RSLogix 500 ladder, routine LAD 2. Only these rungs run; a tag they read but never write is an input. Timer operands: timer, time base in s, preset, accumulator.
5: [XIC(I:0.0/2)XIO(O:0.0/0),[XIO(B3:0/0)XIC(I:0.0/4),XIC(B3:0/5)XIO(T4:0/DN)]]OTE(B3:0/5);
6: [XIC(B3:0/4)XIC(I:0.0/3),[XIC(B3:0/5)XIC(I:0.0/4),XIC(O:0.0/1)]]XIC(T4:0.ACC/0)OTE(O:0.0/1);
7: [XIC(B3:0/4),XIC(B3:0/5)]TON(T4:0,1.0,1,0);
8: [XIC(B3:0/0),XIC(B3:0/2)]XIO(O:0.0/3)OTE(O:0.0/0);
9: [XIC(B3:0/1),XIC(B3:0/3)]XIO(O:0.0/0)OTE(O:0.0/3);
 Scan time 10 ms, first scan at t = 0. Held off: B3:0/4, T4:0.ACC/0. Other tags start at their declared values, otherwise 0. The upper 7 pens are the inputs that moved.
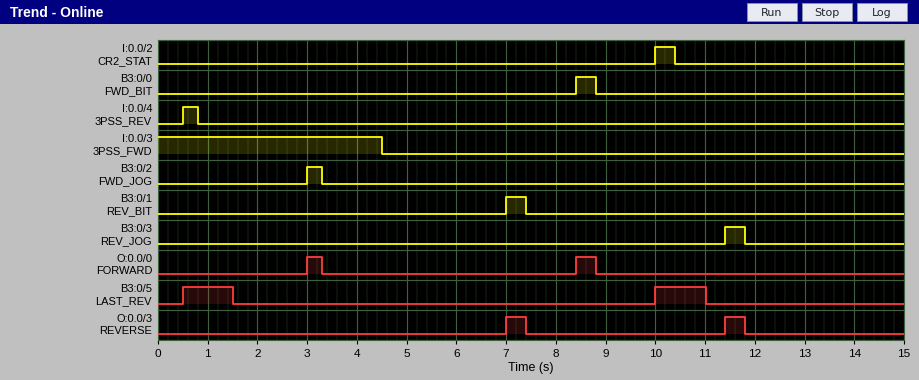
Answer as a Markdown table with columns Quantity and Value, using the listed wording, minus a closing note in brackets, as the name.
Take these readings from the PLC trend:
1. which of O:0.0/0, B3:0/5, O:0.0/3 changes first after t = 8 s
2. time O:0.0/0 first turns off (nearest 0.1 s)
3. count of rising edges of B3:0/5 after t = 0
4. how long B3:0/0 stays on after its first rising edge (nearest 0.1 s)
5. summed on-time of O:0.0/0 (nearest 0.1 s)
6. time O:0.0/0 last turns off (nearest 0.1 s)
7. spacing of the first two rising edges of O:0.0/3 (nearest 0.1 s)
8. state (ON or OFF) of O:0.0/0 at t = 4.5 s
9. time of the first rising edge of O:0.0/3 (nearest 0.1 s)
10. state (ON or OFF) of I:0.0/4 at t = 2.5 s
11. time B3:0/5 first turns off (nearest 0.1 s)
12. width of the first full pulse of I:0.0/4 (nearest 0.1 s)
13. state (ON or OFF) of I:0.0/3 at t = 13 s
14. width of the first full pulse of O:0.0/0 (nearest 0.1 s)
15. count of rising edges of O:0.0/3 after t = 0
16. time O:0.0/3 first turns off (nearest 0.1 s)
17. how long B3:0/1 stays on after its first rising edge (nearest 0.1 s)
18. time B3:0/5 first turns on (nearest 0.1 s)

| Quantity | Value |
|---|---|
| which of O:0.0/0, B3:0/5, O:0.0/3 changes first after t = 8 s | O:0.0/0 |
| time O:0.0/0 first turns off | 3.3 s |
| count of rising edges of B3:0/5 after t = 0 | 2 |
| how long B3:0/0 stays on after its first rising edge | 0.4 s |
| summed on-time of O:0.0/0 | 0.7 s |
| time O:0.0/0 last turns off | 8.8 s |
| spacing of the first two rising edges of O:0.0/3 | 4.4 s |
| state (ON or OFF) of O:0.0/0 at t = 4.5 s | OFF |
| time of the first rising edge of O:0.0/3 | 7.0 s |
| state (ON or OFF) of I:0.0/4 at t = 2.5 s | OFF |
| time B3:0/5 first turns off | 1.5 s |
| width of the first full pulse of I:0.0/4 | 0.3 s |
| state (ON or OFF) of I:0.0/3 at t = 13 s | OFF |
| width of the first full pulse of O:0.0/0 | 0.3 s |
| count of rising edges of O:0.0/3 after t = 0 | 2 |
| time O:0.0/3 first turns off | 7.4 s |
| how long B3:0/1 stays on after its first rising edge | 0.4 s |
| time B3:0/5 first turns on | 0.5 s |
